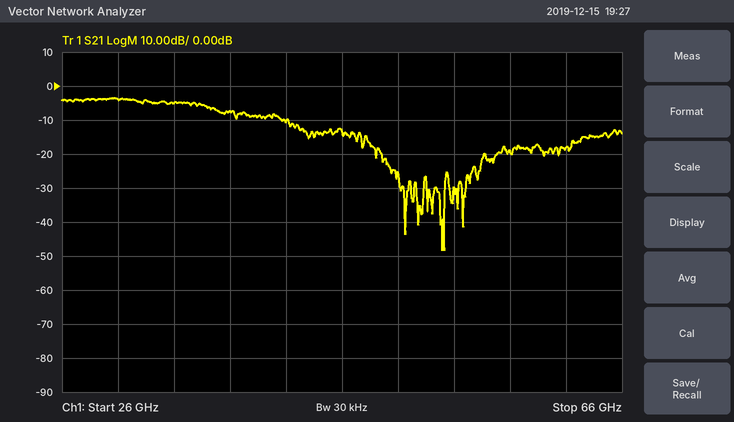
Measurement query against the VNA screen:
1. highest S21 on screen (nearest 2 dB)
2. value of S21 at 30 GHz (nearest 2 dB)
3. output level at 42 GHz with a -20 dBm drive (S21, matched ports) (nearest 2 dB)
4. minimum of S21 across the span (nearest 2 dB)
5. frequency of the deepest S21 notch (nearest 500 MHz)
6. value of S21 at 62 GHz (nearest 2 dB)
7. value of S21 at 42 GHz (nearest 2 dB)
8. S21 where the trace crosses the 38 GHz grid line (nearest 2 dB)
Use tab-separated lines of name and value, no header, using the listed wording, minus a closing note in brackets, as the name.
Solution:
highest S21 on screen	-4 dB
value of S21 at 30 GHz	-4 dB
output level at 42 GHz with a -20 dBm drive (S21, matched ports)	-30 dBm
minimum of S21 across the span	-48 dB
frequency of the deepest S21 notch	53.0 GHz
value of S21 at 62 GHz	-18 dB
value of S21 at 42 GHz	-10 dB
S21 where the trace crosses the 38 GHz grid line	-8 dB
